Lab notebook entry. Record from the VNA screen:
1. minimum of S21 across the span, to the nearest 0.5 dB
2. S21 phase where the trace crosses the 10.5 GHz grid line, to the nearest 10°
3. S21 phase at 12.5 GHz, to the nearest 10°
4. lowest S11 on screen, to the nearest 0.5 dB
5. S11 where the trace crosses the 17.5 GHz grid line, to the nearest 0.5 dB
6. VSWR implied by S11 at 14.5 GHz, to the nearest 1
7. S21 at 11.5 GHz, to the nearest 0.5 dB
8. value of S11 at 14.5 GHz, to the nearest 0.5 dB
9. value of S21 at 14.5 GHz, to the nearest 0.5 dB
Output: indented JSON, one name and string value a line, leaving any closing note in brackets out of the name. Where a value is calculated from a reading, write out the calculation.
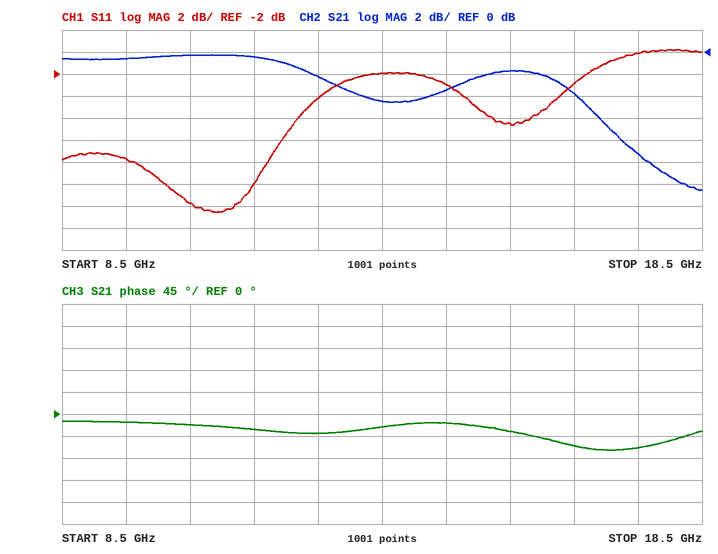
{
  "minimum of S21 across the span, to the nearest 0.5 dB": "-12.5 dB",
  "S21 phase where the trace crosses the 10.5 GHz grid line, to the nearest 10°": "-20°",
  "S21 phase at 12.5 GHz, to the nearest 10°": "-40°",
  "lowest S11 on screen, to the nearest 0.5 dB": "-14.5 dB",
  "S11 where the trace crosses the 17.5 GHz grid line, to the nearest 0.5 dB": "0.0 dB",
  "VSWR implied by S11 at 14.5 GHz, to the nearest 1": "|Γ| = 10^(-3/20) = 0.7079; VSWR = (1 + 0.7079)/(1 − 0.7079) ≈ 6",
  "S21 at 11.5 GHz, to the nearest 0.5 dB": "-0.5 dB",
  "value of S11 at 14.5 GHz, to the nearest 0.5 dB": "-3.0 dB",
  "value of S21 at 14.5 GHz, to the nearest 0.5 dB": "-3.5 dB"
}
